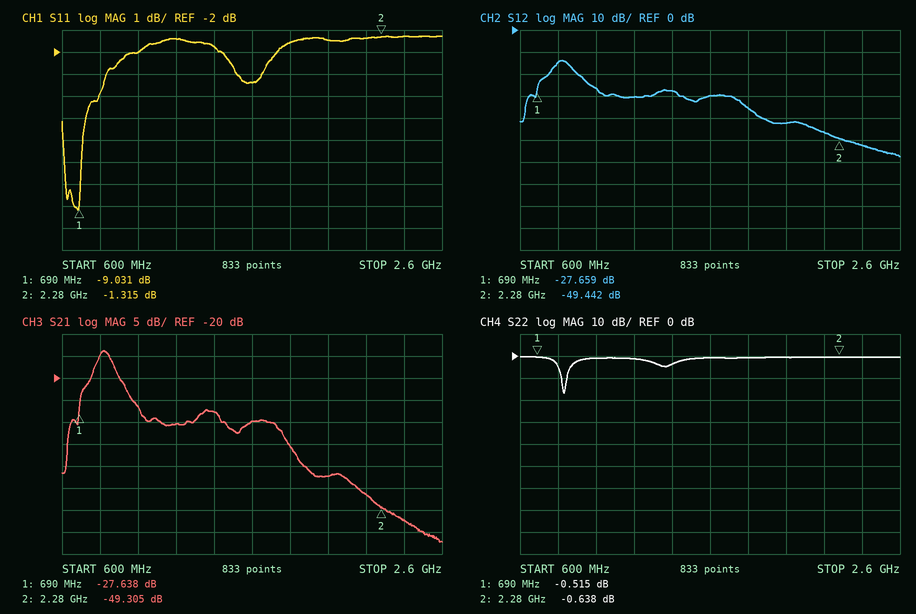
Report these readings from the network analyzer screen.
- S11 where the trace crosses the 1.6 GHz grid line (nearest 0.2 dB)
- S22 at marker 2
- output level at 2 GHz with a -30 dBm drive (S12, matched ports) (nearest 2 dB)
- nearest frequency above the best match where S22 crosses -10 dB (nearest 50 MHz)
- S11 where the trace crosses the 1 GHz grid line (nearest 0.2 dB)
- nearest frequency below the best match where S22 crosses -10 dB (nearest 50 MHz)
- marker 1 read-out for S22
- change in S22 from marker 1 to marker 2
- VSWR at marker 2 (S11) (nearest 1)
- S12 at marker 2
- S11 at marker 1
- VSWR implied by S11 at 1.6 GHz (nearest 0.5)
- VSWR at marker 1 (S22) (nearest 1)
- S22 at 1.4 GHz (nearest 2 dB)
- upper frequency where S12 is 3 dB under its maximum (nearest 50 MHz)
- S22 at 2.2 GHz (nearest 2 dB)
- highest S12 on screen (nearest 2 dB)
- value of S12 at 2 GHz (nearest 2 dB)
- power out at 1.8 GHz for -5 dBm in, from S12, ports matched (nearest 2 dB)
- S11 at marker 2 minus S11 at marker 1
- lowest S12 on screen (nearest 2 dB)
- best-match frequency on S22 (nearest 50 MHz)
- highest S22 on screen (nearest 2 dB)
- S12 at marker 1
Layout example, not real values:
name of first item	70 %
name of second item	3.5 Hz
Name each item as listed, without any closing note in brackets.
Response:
S11 where the trace crosses the 1.6 GHz grid line	-3.4 dB
S22 at marker 2	-0.638 dB
output level at 2 GHz with a -30 dBm drive (S12, matched ports)	-72 dBm
nearest frequency above the best match where S22 crosses -10 dB	850 MHz
S11 where the trace crosses the 1 GHz grid line	-2.0 dB
nearest frequency below the best match where S22 crosses -10 dB	800 MHz
marker 1 read-out for S22	-0.515 dB
change in S22 from marker 1 to marker 2	-0.123 dB
VSWR at marker 2 (S11)	13
S12 at marker 2	-49.442 dB
S11 at marker 1	-9.031 dB
VSWR implied by S11 at 1.6 GHz	5.0
VSWR at marker 1 (S22)	34
S22 at 1.4 GHz	-4 dB
upper frequency where S12 is 3 dB under its maximum	850 MHz
S22 at 2.2 GHz	0 dB
highest S12 on screen	-14 dB
value of S12 at 2 GHz	-42 dB
power out at 1.8 GHz for -5 dBm in, from S12, ports matched	-40 dBm
S11 at marker 2 minus S11 at marker 1	7.716 dB
lowest S12 on screen	-58 dB
best-match frequency on S22	850 MHz
highest S22 on screen	0 dB
S12 at marker 1	-27.659 dB
